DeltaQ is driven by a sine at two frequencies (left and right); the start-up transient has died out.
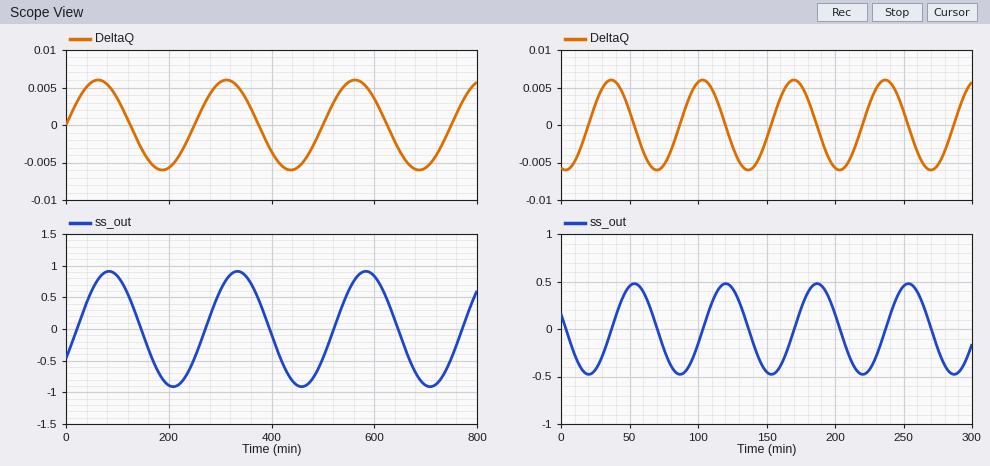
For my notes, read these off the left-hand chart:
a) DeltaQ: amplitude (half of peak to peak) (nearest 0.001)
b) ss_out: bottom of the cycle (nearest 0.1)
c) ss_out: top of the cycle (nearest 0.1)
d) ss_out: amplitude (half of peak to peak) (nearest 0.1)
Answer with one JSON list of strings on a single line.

["0.006", "-0.9", "0.9", "0.9"]
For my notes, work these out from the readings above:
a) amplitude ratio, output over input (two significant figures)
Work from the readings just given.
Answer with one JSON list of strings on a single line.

["150"]
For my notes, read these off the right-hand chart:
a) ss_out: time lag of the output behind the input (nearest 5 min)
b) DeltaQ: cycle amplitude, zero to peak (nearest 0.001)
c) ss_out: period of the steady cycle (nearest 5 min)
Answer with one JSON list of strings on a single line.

["15 min", "0.006", "65 min"]
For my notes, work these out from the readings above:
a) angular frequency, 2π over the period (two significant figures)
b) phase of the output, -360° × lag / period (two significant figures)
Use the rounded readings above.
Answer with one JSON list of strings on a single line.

["0.097 rad/min", "-83°"]
